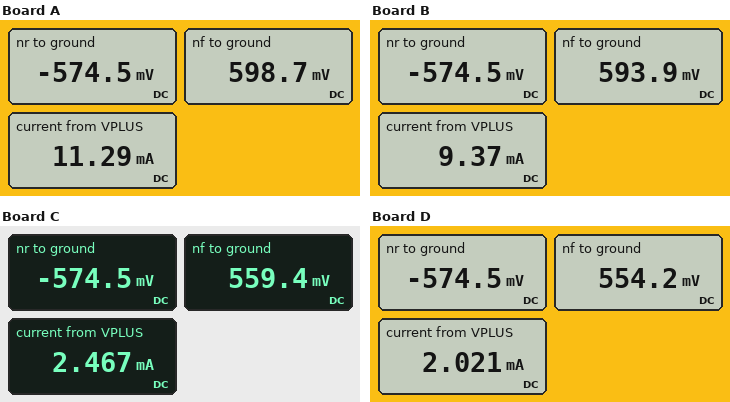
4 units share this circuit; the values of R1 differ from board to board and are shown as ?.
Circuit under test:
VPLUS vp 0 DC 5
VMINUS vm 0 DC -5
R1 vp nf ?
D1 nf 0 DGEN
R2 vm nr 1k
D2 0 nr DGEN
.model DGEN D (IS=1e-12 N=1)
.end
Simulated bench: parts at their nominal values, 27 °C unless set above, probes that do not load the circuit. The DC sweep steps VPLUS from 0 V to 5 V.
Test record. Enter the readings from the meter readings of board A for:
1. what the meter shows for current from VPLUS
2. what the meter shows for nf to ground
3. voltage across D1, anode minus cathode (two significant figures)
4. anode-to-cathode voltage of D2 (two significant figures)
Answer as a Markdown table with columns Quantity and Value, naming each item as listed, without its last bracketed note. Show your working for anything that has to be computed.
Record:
| Quantity | Value |
|---|---|
| what the meter shows for current from VPLUS | 11.29 mA |
| what the meter shows for nf to ground | 598.7 mV |
| voltage across D1, anode minus cathode | 598.7 mV = 600 mV |
| anode-to-cathode voltage of D2 | 0 V - (-574.5 mV) = 570 mV |
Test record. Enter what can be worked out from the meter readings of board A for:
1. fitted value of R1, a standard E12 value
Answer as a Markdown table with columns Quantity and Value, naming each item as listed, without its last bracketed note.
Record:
| Quantity | Value |
|---|---|
| fitted value of R1, a standard E12 value | 390 Ω |
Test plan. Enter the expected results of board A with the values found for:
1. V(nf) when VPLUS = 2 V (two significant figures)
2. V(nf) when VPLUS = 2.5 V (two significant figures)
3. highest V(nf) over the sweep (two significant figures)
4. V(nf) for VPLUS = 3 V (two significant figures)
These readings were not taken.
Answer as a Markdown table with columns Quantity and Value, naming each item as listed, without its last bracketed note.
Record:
| Quantity | Value |
|---|---|
| V(nf) when VPLUS = 2 V | 570 mV |
| V(nf) when VPLUS = 2.5 V | 580 mV |
| highest V(nf) over the sweep | 600 mV |
| V(nf) for VPLUS = 3 V | 580 mV |
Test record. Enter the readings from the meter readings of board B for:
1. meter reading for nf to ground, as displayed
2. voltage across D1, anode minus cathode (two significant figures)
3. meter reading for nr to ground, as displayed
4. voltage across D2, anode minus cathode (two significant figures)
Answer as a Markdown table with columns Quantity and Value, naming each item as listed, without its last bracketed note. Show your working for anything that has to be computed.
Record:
| Quantity | Value |
|---|---|
| meter reading for nf to ground, as displayed | 593.9 mV |
| voltage across D1, anode minus cathode | 593.9 mV = 590 mV |
| meter reading for nr to ground, as displayed | -574.5 mV |
| voltage across D2, anode minus cathode | 0 V - (-574.5 mV) = 570 mV |
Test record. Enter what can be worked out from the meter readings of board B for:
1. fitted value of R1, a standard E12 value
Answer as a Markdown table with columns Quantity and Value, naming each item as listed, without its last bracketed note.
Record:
| Quantity | Value |
|---|---|
| fitted value of R1, a standard E12 value | 470 Ω |
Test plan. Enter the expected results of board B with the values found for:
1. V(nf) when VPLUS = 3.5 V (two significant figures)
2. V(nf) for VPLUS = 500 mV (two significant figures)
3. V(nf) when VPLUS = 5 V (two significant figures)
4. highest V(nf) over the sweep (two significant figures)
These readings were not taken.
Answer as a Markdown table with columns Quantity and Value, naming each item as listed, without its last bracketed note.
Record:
| Quantity | Value |
|---|---|
| V(nf) when VPLUS = 3.5 V | 580 mV |
| V(nf) for VPLUS = 500 mV | 470 mV |
| V(nf) when VPLUS = 5 V | 590 mV |
| highest V(nf) over the sweep | 590 mV |
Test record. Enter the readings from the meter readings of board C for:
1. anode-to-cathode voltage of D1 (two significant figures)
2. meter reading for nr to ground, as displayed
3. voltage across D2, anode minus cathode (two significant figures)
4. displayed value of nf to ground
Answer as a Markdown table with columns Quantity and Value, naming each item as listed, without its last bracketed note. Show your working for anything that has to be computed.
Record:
| Quantity | Value |
|---|---|
| anode-to-cathode voltage of D1 | 559.4 mV = 560 mV |
| meter reading for nr to ground, as displayed | -574.5 mV |
| voltage across D2, anode minus cathode | 0 V - (-574.5 mV) = 570 mV |
| displayed value of nf to ground | 559.4 mV |
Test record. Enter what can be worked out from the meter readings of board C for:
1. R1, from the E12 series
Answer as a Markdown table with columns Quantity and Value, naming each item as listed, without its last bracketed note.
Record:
| Quantity | Value |
|---|---|
| R1, from the E12 series | 1.8 kΩ |
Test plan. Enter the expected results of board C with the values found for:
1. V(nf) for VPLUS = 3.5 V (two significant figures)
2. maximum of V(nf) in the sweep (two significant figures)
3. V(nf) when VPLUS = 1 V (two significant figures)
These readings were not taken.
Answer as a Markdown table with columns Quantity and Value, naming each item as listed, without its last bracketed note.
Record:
| Quantity | Value |
|---|---|
| V(nf) for VPLUS = 3.5 V | 550 mV |
| maximum of V(nf) in the sweep | 560 mV |
| V(nf) when VPLUS = 1 V | 500 mV |
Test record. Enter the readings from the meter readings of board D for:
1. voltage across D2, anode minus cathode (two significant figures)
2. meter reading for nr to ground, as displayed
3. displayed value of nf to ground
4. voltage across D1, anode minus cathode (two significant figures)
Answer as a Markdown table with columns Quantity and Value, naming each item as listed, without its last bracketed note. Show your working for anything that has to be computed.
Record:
| Quantity | Value |
|---|---|
| voltage across D2, anode minus cathode | 0 V - (-574.5 mV) = 570 mV |
| meter reading for nr to ground, as displayed | -574.5 mV |
| displayed value of nf to ground | 554.2 mV |
| voltage across D1, anode minus cathode | 554.2 mV = 550 mV |
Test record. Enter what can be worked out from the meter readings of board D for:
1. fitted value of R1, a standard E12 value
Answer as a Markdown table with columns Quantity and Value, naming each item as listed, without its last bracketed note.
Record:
| Quantity | Value |
|---|---|
| fitted value of R1, a standard E12 value | 2.2 kΩ |
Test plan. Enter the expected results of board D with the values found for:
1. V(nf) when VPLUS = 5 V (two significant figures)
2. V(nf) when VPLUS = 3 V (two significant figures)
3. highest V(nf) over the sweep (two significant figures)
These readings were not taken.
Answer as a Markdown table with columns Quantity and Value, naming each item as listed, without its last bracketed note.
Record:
| Quantity | Value |
|---|---|
| V(nf) when VPLUS = 5 V | 550 mV |
| V(nf) when VPLUS = 3 V | 540 mV |
| highest V(nf) over the sweep | 550 mV |
